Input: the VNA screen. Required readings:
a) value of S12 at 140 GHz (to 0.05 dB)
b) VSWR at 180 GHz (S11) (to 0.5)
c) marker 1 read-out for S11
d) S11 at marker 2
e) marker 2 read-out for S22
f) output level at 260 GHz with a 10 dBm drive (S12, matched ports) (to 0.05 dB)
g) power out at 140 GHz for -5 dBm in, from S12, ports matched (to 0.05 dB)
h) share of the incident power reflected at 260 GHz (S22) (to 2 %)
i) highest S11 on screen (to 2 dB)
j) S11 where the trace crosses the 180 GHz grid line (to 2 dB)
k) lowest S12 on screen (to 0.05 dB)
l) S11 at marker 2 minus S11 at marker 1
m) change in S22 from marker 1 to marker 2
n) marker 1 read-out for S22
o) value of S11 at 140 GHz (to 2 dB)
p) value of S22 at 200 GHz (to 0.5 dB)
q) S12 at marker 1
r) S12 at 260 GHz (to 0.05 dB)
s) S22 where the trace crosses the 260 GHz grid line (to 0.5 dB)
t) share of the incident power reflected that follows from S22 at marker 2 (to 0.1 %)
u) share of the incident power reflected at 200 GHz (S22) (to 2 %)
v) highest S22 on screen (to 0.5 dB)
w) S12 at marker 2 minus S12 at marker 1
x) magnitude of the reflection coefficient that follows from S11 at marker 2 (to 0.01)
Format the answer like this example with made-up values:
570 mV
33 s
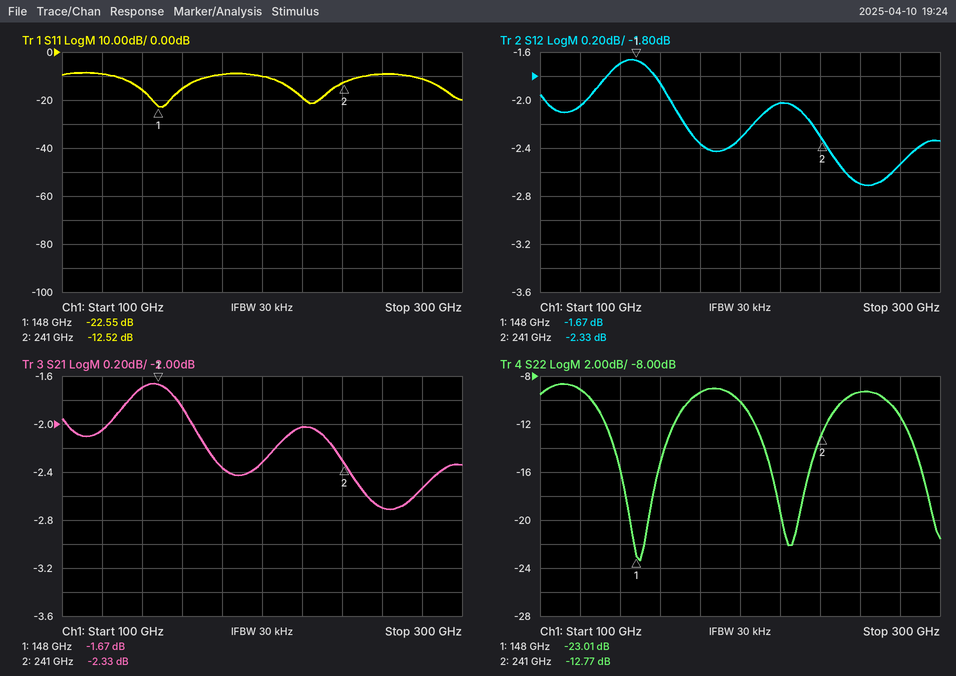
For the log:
-1.70 dB
2.0
-22.55 dB
-12.52 dB
-12.77 dB
7.30 dBm
-6.70 dBm
12 %
-8 dB
-10 dB
-2.70 dB
10.03 dB
10.24 dB
-23.01 dB
-16 dB
-10.0 dB
-1.67 dB
-2.70 dB
-9.5 dB
5.3 %
10 %
-8.5 dB
-0.66 dB
0.24
